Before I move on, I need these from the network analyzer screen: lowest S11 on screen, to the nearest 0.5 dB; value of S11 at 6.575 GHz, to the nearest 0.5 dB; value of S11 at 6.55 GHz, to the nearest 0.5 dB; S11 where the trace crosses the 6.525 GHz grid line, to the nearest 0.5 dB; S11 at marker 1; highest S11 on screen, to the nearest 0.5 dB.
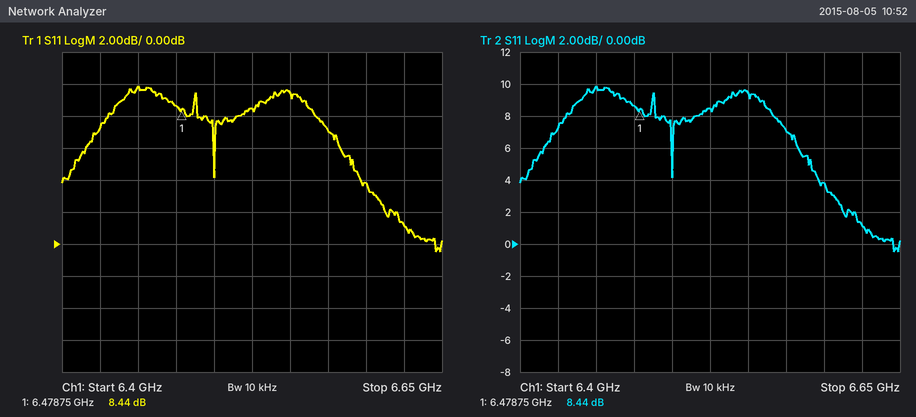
-0.5 dB
7.0 dB
9.5 dB
8.5 dB
8.44 dB
10.0 dB
